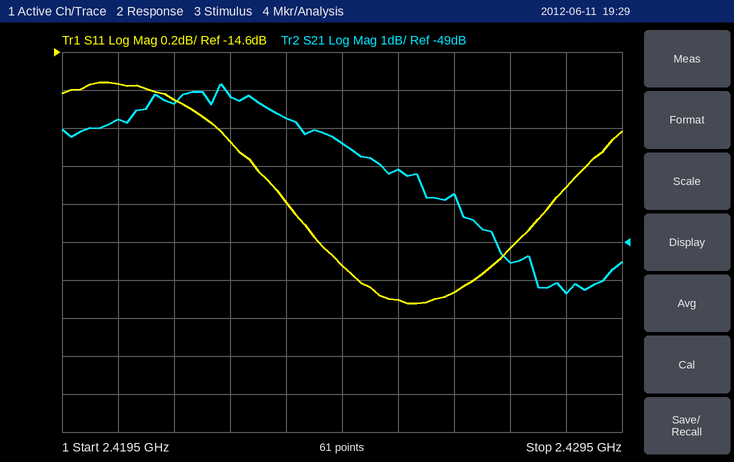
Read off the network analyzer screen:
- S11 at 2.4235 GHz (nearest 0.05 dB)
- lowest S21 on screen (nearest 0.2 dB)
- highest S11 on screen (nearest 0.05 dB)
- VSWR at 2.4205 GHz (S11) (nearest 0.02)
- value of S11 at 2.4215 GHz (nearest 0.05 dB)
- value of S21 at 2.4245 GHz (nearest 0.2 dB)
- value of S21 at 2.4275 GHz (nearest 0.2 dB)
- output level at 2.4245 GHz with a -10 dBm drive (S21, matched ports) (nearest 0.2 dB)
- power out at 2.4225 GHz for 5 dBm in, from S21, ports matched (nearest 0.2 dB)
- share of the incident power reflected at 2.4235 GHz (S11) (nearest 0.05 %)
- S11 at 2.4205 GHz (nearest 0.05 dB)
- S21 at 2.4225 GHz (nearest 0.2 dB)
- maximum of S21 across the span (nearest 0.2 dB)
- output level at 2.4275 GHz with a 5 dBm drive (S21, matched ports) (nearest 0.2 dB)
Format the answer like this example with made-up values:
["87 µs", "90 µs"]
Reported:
["-15.40 dB", "-50.4 dB", "-14.75 dB", "1.44", "-14.85 dB", "-46.4 dB", "-49.6 dB", "-56.4 dBm", "-40.2 dBm", "2.90 %", "-14.75 dB", "-45.2 dB", "-44.8 dB", "-44.6 dBm"]
